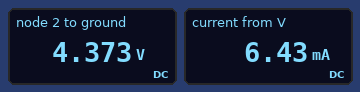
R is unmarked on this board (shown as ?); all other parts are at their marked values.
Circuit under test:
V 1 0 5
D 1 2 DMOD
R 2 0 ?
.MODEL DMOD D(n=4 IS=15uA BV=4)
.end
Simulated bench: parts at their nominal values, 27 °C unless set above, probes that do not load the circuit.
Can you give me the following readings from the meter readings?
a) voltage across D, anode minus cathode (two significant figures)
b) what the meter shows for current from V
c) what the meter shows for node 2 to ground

630 mV
6.43 mA
4.373 V
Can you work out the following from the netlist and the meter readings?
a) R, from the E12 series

680 Ω
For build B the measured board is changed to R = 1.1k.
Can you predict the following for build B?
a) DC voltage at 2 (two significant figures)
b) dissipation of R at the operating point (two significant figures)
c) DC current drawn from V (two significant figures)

4.4 V
18 mW
4.0 mA
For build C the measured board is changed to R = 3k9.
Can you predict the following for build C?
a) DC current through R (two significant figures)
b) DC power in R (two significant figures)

1.2 mA
5.3 mW
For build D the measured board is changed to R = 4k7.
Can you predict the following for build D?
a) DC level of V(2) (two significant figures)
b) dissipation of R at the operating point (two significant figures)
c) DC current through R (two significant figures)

4.6 V
4.4 mW
970 µA
